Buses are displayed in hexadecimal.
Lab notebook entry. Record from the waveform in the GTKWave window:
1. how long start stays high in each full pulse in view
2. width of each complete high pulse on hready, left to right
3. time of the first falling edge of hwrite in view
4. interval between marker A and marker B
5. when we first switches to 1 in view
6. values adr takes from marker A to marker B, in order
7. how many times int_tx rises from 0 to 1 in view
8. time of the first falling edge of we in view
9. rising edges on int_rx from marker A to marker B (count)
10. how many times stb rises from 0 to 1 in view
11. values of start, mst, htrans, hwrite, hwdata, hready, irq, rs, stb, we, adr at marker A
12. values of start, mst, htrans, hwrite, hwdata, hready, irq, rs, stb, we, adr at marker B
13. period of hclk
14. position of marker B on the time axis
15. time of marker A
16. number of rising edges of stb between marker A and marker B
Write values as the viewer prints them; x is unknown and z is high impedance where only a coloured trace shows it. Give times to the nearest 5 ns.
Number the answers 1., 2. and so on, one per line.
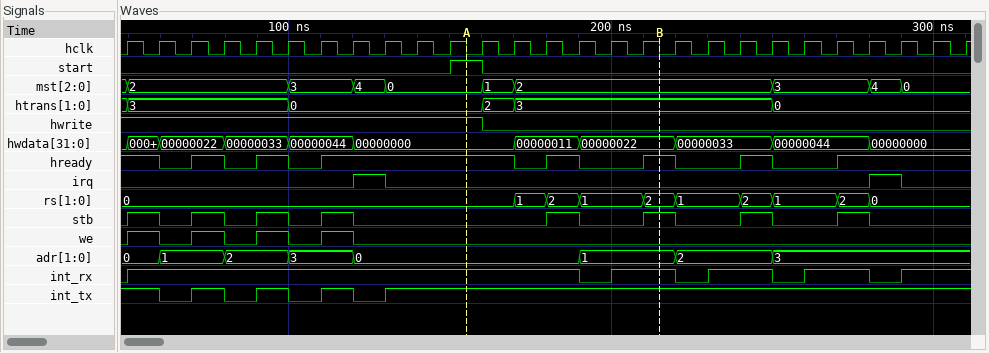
1. 10 ns
2. 10 ns, 10 ns, 60 ns, 10 ns, 10 ns, 10 ns
3. 160 ns
4. 60 ns
5. 50 ns
6. 0, 1
7. 4
8. 60 ns
9. 1
10. 8
11. start=1, mst=0, htrans=0, hwrite=1, hwdata=00000000, hready=1, irq=0, rs=0, stb=0, we=0, adr=0
12. start=0, mst=2, htrans=3, hwrite=0, hwdata=00000022, hready=1, irq=0, rs=2, stb=1, we=0, adr=1
13. 10 ns
14. 215 ns
15. 155 ns
16. 2
